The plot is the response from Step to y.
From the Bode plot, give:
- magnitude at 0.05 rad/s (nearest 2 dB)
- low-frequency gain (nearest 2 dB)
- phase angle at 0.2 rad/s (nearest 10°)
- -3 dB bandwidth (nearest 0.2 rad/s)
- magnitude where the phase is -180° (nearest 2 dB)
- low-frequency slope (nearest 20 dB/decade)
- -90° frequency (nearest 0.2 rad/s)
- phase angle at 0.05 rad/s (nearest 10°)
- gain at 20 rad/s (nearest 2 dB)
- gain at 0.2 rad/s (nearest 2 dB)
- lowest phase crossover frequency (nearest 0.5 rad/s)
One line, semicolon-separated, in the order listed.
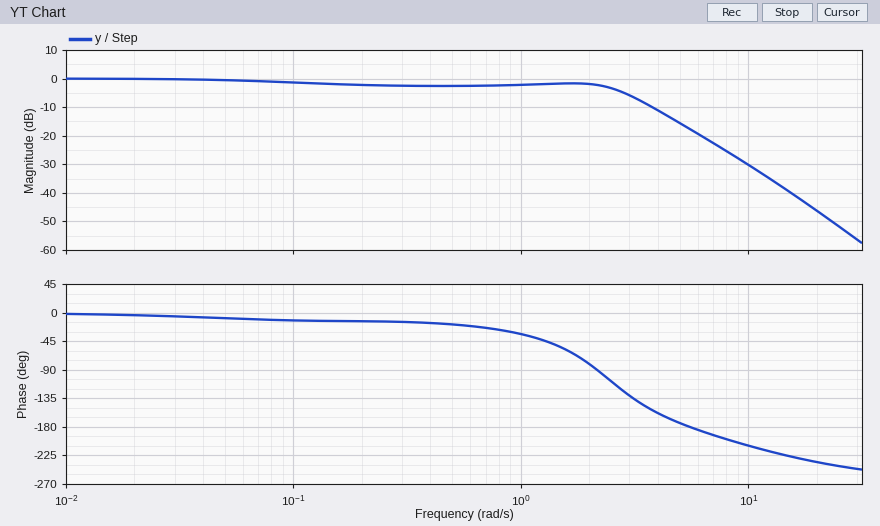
0 dB; 0 dB; -10°; 2.4 rad/s; -18 dB; 0 dB/decade; 2.2 rad/s; -10°; -46 dB; -2 dB; 5.5 rad/s
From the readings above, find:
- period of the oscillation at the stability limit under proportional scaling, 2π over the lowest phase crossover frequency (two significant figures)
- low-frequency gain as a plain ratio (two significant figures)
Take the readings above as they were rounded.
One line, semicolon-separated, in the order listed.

1.1 s; 1.0
